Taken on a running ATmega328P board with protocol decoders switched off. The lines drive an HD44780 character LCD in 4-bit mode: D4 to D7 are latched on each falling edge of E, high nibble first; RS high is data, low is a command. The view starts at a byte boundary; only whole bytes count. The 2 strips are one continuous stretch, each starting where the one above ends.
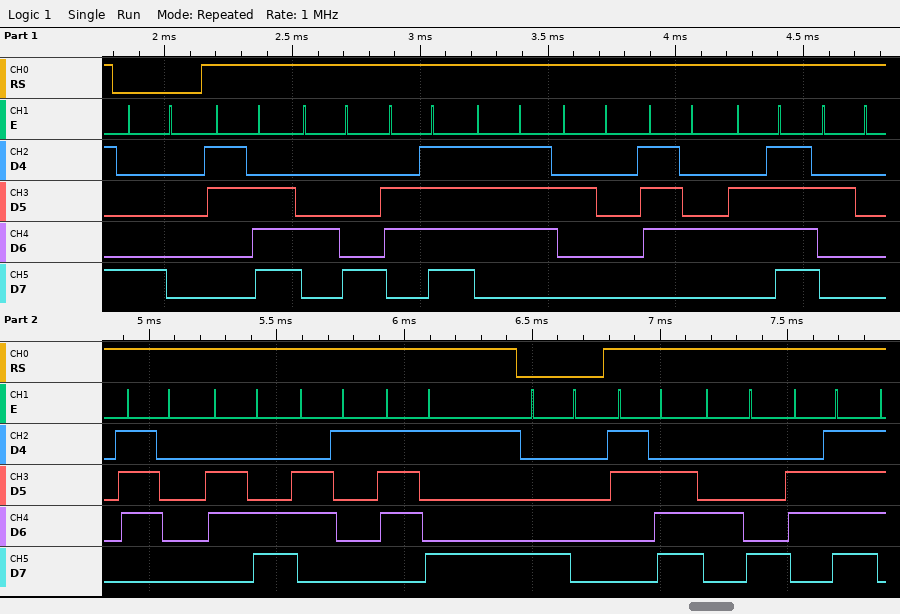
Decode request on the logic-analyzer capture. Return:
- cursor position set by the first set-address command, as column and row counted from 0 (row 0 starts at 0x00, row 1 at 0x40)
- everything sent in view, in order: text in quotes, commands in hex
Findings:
column 0, row 0
0x80 ">How to play" 0x80 ">Ho"
